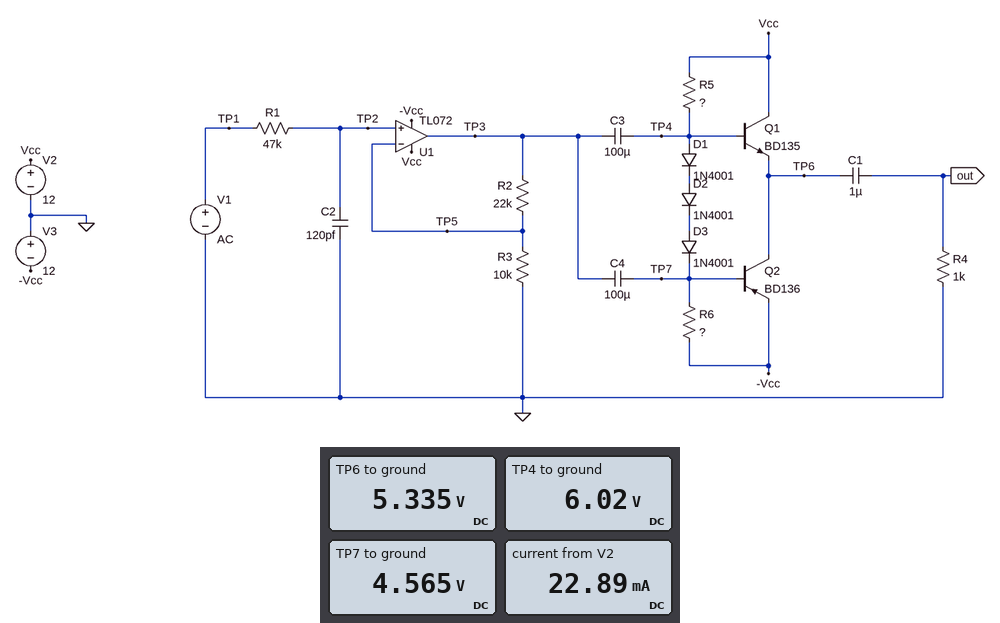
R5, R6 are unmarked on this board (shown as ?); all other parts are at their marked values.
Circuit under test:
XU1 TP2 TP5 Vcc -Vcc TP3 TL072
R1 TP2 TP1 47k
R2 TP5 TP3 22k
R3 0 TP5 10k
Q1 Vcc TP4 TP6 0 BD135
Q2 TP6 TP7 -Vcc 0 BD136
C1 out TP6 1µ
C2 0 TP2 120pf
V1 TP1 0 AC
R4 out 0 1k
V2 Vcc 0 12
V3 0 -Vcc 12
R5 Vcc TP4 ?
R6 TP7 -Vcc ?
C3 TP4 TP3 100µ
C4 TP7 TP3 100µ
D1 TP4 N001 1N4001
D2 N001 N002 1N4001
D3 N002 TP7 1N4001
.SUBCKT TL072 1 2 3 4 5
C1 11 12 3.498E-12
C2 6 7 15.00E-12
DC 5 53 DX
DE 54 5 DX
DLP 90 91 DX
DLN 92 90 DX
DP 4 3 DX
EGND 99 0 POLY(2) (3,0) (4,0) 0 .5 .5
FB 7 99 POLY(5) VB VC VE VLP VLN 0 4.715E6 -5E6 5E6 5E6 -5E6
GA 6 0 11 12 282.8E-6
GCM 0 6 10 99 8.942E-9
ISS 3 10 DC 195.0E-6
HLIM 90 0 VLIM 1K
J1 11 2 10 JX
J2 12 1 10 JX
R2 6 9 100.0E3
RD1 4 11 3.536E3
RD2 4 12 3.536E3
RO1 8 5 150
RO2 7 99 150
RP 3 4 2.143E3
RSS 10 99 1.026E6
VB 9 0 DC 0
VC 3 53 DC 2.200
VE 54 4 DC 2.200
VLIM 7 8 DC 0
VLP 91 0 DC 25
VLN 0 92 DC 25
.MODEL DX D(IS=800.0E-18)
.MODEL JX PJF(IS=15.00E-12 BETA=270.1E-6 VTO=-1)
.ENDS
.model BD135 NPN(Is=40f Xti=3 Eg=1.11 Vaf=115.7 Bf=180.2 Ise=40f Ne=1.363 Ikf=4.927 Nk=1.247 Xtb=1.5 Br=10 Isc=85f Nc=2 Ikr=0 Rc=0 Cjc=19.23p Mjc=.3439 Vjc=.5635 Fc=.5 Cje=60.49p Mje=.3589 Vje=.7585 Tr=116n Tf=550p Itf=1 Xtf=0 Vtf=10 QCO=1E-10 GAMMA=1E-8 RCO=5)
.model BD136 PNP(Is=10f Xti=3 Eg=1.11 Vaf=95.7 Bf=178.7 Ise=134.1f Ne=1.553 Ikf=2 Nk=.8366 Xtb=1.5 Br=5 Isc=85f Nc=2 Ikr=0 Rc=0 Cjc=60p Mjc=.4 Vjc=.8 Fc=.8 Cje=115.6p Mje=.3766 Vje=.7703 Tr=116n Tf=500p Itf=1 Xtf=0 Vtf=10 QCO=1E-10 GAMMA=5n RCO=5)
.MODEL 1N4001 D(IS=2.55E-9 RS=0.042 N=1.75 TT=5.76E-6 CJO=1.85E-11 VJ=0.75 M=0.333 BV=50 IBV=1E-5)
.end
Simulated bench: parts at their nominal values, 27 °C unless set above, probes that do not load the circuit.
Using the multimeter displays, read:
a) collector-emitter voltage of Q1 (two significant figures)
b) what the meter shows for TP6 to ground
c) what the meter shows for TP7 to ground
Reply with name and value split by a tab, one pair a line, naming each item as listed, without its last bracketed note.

collector-emitter voltage of Q1	6.7 V
what the meter shows for TP6 to ground	5.335 V
what the meter shows for TP7 to ground	4.565 V
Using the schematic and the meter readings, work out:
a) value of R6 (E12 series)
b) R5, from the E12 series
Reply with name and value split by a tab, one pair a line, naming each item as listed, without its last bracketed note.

value of R6	8.2 kΩ
R5, from the E12 series	33 kΩ
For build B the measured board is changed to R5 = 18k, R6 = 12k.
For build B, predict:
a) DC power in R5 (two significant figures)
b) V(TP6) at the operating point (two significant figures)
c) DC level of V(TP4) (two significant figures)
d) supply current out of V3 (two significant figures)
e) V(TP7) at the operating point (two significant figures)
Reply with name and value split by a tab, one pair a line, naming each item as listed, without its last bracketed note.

DC power in R5	430 µW
V(TP6) at the operating point	8.5 V
DC level of V(TP4)	9.2 V
supply current out of V3	21 mA
V(TP7) at the operating point	7.8 V
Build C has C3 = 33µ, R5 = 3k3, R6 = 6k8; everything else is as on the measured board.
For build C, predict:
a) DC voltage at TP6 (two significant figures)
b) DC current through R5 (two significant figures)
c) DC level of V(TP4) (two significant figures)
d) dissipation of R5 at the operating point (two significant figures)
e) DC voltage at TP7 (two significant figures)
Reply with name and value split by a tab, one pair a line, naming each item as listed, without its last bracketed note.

DC voltage at TP6	10 V
DC current through R5	280 µA
DC level of V(TP4)	11 V
dissipation of R5 at the operating point	260 µW
DC voltage at TP7	9.6 V
